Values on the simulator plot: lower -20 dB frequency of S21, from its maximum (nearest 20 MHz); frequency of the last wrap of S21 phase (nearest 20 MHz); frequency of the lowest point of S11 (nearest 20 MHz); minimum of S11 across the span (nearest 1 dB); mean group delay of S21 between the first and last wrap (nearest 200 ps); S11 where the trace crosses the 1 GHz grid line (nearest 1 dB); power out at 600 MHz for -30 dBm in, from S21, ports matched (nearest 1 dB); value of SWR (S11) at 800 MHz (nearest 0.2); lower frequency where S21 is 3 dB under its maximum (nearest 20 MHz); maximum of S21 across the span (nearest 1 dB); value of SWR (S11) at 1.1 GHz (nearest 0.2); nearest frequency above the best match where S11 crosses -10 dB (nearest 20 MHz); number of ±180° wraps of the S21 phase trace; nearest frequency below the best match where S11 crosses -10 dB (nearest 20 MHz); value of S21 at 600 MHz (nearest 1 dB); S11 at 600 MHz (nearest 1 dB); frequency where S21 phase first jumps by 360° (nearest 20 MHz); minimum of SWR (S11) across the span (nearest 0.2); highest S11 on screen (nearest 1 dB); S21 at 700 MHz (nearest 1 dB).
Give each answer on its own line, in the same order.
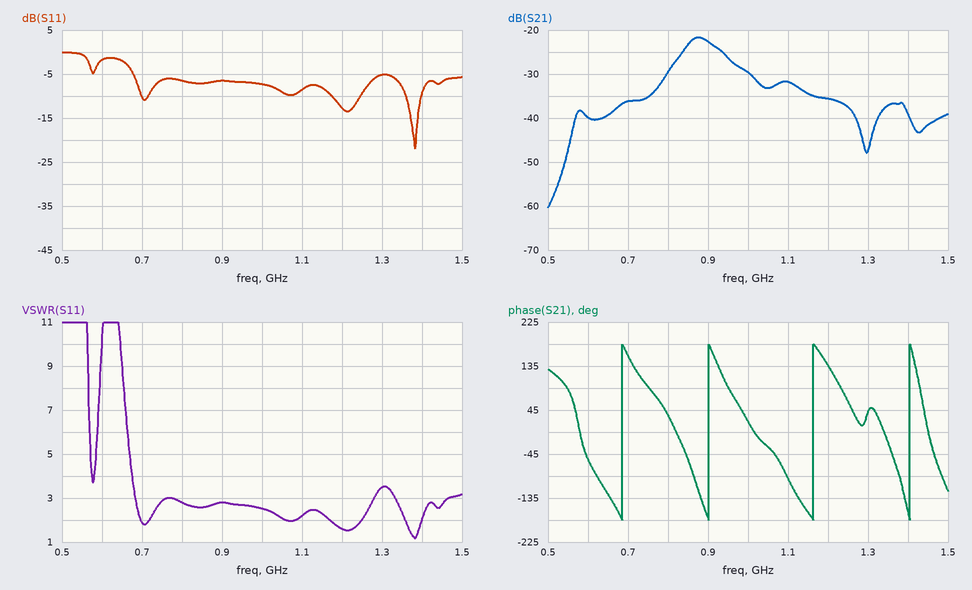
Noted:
560 MHz
1.40 GHz
1.38 GHz
-22 dB
4.2 ns
-7 dB
-70 dBm
2.8
840 MHz
-22 dB
2.2
1.40 GHz
4
1.36 GHz
-40 dB
-2 dB
680 MHz
1.2
0 dB
-36 dB
